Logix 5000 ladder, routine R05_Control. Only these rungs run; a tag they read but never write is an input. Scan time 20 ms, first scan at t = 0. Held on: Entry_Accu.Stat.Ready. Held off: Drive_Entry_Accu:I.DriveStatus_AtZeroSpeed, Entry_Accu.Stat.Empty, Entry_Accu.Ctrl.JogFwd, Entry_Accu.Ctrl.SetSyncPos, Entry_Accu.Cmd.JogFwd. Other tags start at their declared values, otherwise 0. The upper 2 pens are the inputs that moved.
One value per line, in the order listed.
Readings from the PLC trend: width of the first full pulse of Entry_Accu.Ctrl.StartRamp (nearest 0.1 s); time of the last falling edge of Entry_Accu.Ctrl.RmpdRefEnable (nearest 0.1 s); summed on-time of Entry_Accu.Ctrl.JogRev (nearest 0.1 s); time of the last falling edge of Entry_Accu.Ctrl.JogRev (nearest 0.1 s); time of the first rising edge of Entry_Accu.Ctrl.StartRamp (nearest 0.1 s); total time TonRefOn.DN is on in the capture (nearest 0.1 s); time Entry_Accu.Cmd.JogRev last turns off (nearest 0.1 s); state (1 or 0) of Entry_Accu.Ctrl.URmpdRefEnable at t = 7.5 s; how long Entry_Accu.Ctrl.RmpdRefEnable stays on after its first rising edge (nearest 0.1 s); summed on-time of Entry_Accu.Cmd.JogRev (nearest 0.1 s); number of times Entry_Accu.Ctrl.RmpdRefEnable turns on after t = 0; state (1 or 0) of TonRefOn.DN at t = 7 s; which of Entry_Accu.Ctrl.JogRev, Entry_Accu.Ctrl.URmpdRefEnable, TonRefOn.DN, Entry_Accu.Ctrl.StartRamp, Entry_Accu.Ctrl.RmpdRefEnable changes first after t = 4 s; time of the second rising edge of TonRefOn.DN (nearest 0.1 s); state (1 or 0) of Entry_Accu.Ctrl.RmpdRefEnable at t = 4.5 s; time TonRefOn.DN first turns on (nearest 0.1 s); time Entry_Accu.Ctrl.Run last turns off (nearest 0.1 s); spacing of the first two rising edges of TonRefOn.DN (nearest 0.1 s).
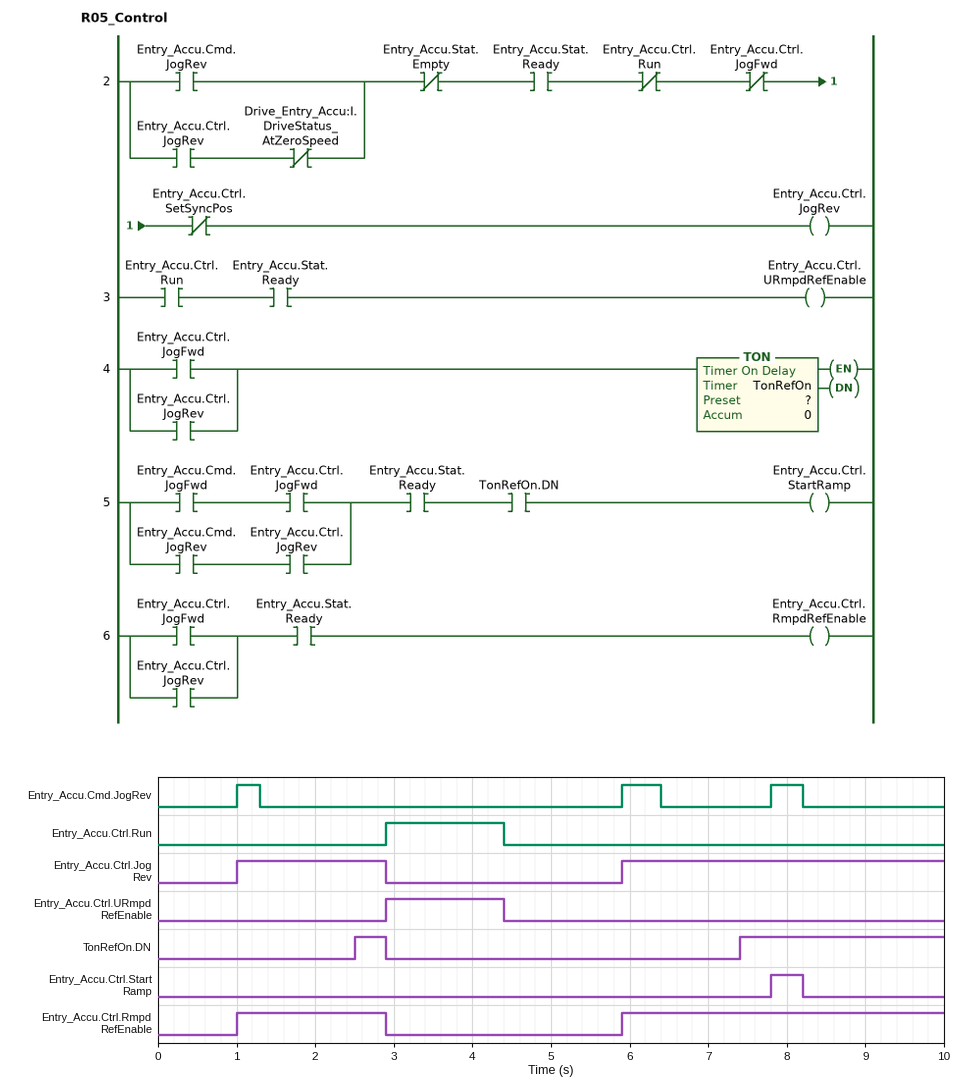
0.4 s
2.9 s
6.0 s
2.9 s
7.8 s
3.0 s
8.2 s
0
1.9 s
1.2 s
2
0
Entry_Accu.Ctrl.URmpdRefEnable
7.4 s
0
2.5 s
4.4 s
4.9 s
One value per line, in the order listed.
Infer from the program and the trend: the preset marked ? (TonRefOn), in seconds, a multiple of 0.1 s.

1.5 s
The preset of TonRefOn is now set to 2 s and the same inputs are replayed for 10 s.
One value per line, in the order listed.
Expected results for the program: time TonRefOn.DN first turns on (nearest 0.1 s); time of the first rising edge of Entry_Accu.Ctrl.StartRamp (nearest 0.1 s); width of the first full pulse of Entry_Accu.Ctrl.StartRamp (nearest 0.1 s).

7.9 s
7.9 s
0.3 s
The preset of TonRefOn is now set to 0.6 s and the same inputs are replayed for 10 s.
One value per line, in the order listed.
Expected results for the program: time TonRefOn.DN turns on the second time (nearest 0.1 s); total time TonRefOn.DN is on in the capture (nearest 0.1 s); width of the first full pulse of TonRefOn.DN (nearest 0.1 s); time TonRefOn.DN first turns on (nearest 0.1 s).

6.5 s
4.8 s
1.3 s
1.6 s
